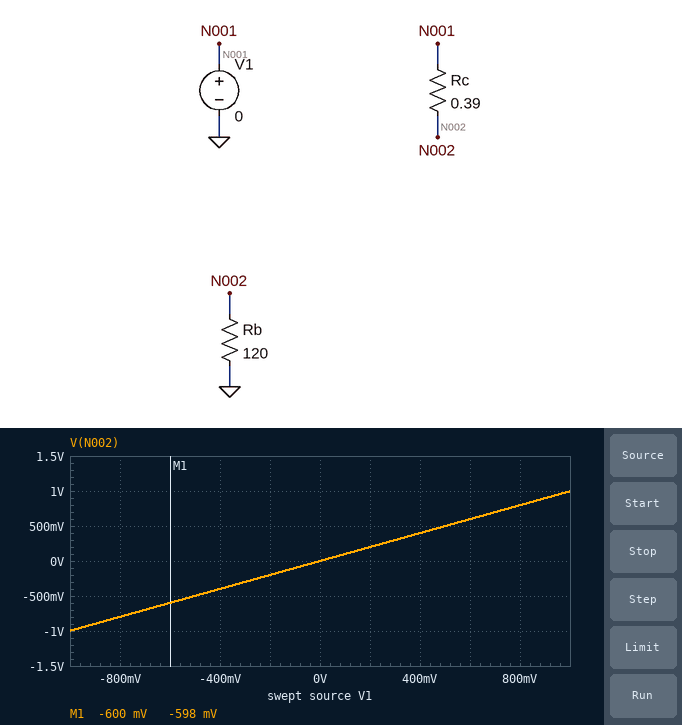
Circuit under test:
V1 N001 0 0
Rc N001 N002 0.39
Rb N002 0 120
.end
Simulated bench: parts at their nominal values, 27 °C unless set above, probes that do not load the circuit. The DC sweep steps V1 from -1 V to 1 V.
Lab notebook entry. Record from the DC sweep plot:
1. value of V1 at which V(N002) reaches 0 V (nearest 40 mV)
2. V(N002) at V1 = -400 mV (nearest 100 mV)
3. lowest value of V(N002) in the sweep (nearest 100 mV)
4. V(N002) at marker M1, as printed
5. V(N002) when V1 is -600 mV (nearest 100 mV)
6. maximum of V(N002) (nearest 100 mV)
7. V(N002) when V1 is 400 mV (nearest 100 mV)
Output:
0 V
-400 mV
-1.0 V
-598 mV
-600 mV
1.0 V
400 mV
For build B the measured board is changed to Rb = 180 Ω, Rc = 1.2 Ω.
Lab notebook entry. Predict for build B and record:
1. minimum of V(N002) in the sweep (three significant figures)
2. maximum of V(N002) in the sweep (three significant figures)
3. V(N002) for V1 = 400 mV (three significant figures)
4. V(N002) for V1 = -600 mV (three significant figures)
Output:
-993 mV
993 mV
397 mV
-596 mV
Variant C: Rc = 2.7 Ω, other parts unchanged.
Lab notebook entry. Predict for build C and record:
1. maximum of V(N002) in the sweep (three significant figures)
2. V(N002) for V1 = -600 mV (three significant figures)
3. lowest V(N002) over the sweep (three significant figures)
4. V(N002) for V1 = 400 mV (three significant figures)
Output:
978 mV
-587 mV
-978 mV
391 mV
